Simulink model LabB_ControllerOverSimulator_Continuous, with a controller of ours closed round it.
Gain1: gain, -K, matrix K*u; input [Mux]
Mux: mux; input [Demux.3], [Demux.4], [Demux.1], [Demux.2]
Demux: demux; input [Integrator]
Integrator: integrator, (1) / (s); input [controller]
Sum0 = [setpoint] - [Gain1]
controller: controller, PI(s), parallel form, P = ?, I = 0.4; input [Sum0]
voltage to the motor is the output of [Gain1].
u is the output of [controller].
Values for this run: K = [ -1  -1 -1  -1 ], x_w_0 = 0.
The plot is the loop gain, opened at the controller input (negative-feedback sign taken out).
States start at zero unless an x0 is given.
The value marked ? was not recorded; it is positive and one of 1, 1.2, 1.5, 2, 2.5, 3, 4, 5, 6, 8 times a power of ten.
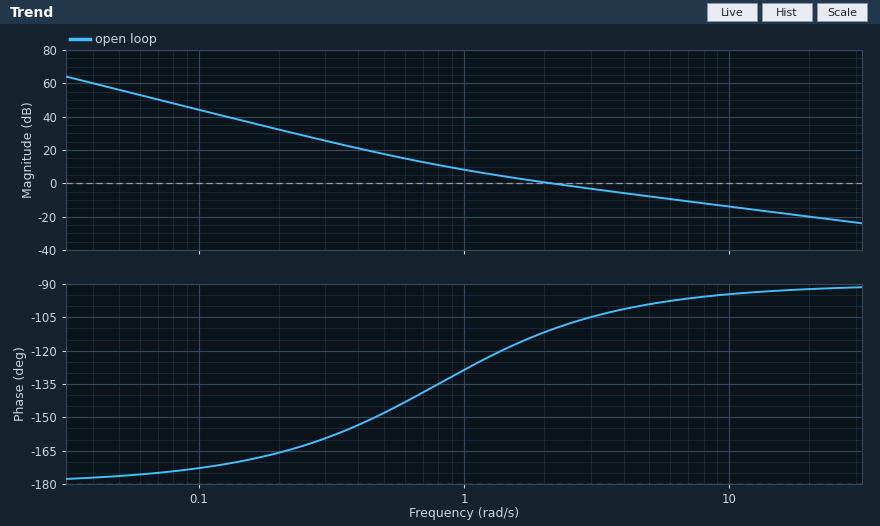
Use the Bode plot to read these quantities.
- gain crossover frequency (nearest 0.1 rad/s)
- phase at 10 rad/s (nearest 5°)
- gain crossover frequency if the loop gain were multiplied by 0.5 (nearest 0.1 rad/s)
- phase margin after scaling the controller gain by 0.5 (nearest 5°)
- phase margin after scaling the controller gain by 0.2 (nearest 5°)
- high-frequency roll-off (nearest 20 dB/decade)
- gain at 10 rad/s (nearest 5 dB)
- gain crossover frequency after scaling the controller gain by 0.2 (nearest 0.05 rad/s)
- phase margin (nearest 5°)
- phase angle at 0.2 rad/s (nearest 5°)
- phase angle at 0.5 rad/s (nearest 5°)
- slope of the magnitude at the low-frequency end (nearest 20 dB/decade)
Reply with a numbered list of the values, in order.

1. 2.1 rad/s
2. -95°
3. 1.2 rad/s
4. 55°
5. 40°
6. -20 dB/decade
7. -15 dB
8. 0.65 rad/s
9. 70°
10. -165°
11. -150°
12. -40 dB/decade
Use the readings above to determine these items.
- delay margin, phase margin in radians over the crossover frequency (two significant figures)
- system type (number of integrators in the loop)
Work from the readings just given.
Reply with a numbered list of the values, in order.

1. 0.58 s
2. 2
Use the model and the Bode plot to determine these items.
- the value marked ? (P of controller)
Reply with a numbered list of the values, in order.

1. 0.5
